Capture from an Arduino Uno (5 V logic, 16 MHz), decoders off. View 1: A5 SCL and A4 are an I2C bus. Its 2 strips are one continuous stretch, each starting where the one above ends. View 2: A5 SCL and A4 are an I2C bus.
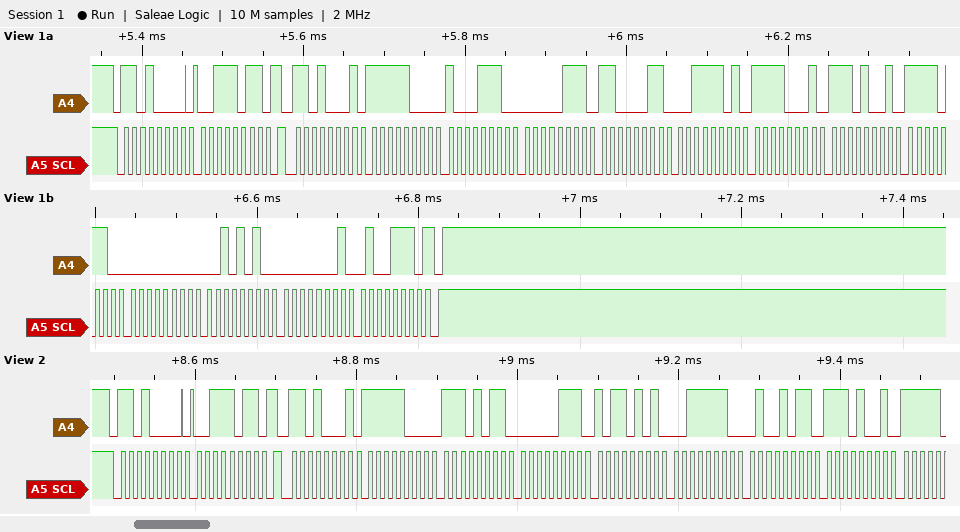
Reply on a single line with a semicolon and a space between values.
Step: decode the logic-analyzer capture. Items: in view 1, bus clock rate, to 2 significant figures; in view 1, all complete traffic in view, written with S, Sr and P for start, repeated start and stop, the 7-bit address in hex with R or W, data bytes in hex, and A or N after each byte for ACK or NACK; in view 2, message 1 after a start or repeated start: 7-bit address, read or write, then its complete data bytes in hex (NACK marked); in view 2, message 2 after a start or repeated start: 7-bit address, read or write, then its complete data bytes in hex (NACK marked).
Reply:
100 kHz; S 68W A 3B A Sr 68R A F8 A 8E A 07 A C3 A 3D A F1 A E9 A F6 A 00 A 2A A 01 A 4E N P; 0x68 write: 3B; 0x68 read: F8 EB 07 B5 3E 4B E9
